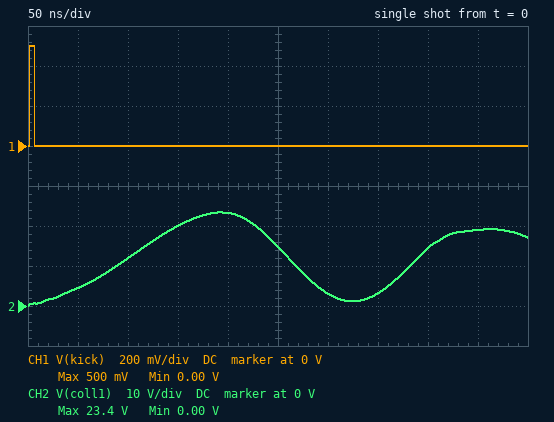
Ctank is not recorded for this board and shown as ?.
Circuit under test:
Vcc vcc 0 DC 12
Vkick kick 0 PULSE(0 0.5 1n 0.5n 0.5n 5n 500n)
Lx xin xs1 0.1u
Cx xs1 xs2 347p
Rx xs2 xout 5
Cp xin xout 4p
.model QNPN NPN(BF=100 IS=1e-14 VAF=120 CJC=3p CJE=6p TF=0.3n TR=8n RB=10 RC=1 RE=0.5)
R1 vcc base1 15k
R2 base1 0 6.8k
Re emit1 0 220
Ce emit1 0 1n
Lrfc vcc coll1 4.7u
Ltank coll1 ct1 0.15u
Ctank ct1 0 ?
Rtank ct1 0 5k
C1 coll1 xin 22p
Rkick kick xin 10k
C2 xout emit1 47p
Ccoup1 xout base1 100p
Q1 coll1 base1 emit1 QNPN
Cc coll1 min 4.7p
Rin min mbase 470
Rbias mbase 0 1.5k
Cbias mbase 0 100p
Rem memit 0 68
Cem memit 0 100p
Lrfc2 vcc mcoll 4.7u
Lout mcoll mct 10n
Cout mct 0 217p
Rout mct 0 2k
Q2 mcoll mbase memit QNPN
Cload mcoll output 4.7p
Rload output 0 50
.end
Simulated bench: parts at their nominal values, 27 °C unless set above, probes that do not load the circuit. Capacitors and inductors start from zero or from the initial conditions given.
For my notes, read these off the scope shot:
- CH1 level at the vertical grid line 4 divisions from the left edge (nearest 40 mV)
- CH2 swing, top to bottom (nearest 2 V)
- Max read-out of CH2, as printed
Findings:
0 V
24 V
23.4 V
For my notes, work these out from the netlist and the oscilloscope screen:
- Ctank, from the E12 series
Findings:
330 pF
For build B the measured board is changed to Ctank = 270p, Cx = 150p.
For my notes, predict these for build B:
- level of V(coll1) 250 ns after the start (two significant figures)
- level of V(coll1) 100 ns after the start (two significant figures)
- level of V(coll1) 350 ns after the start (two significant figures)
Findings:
11 V
13 V
8.4 V
